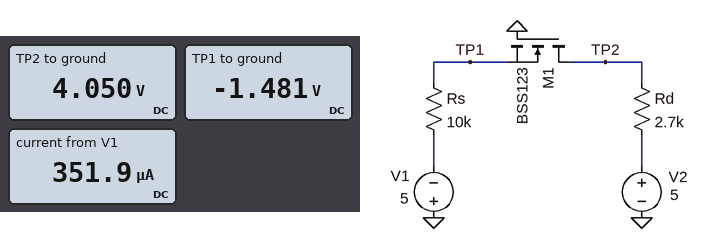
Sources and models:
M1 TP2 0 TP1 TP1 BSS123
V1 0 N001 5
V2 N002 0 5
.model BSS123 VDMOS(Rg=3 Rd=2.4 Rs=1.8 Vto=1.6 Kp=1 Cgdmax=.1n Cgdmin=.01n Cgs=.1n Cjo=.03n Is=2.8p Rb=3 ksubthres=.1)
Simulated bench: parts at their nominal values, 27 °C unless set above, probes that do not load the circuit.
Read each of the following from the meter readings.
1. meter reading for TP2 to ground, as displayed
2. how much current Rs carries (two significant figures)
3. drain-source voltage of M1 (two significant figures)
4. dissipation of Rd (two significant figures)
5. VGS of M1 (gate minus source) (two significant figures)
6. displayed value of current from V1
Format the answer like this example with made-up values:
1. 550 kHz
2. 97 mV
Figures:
1. 4.050 V
2. 350 µA
3. 5.5 V
4. 330 µW
5. 1.5 V
6. 351.9 µA
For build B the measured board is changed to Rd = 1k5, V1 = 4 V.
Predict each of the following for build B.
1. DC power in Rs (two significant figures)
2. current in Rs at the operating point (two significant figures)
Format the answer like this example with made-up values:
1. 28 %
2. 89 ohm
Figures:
1. 640 µW
2. 250 µA
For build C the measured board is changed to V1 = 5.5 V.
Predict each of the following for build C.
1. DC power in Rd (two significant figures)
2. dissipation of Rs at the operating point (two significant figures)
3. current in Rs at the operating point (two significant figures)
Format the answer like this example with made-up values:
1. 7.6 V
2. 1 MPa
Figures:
1. 430 µW
2. 1.6 mW
3. 400 µA
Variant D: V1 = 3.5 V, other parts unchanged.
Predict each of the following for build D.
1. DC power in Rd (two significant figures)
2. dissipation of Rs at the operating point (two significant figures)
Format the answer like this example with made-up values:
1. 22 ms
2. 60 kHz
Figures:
1. 110 µW
2. 420 µW
